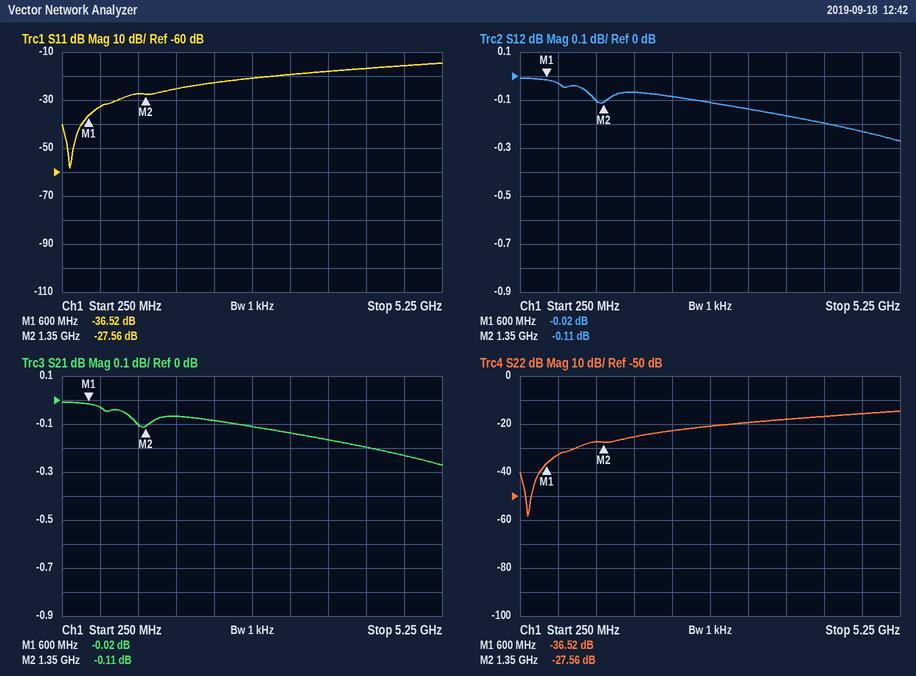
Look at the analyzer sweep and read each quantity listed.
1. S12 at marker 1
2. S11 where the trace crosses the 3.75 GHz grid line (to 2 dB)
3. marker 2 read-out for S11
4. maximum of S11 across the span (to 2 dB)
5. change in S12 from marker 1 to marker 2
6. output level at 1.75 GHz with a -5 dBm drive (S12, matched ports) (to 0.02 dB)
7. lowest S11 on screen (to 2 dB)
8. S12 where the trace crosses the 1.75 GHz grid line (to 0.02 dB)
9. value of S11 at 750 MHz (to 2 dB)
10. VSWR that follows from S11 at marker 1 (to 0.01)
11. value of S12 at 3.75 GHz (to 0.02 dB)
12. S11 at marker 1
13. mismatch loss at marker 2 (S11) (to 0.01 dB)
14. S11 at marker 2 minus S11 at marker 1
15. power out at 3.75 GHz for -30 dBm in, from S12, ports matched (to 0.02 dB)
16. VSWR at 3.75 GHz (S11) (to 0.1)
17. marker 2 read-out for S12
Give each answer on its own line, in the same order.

-0.02 dB
-18 dB
-27.56 dB
-14 dB
-0.09 dB
-5.06 dBm
-58 dB
-0.06 dB
-32 dB
1.03
-0.16 dB
-36.52 dB
0.01 dB
8.96 dB
-30.16 dBm
1.3
-0.11 dB
